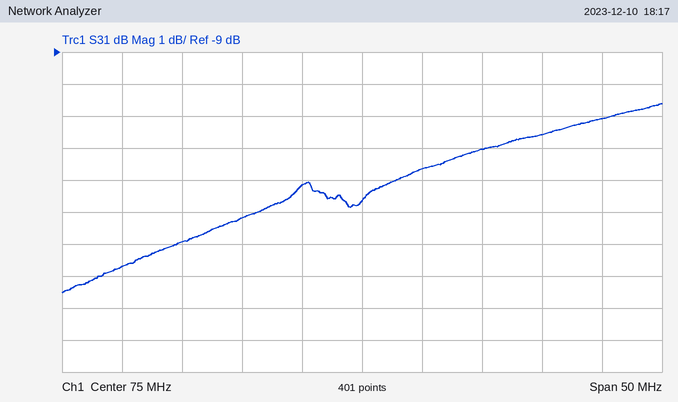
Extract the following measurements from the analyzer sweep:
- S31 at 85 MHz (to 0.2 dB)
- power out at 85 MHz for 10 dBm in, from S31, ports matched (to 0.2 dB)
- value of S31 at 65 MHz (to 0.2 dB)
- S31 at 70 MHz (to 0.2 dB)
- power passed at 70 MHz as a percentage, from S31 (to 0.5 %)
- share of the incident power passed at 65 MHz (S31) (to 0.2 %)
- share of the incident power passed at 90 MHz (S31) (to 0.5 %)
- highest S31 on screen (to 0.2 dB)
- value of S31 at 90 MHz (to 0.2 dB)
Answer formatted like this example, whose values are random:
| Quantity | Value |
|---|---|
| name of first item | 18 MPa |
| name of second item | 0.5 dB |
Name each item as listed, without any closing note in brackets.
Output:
| Quantity | Value |
|---|---|
| S31 at 85 MHz | -12.0 dB |
| power out at 85 MHz for 10 dBm in, from S31, ports matched | -2.0 dBm |
| value of S31 at 65 MHz | -14.2 dB |
| S31 at 70 MHz | -13.2 dB |
| power passed at 70 MHz as a percentage, from S31 | 5.0 % |
| share of the incident power passed at 65 MHz (S31) | 3.8 % |
| share of the incident power passed at 90 MHz (S31) | 7.0 % |
| highest S31 on screen | -10.6 dB |
| value of S31 at 90 MHz | -11.6 dB |
